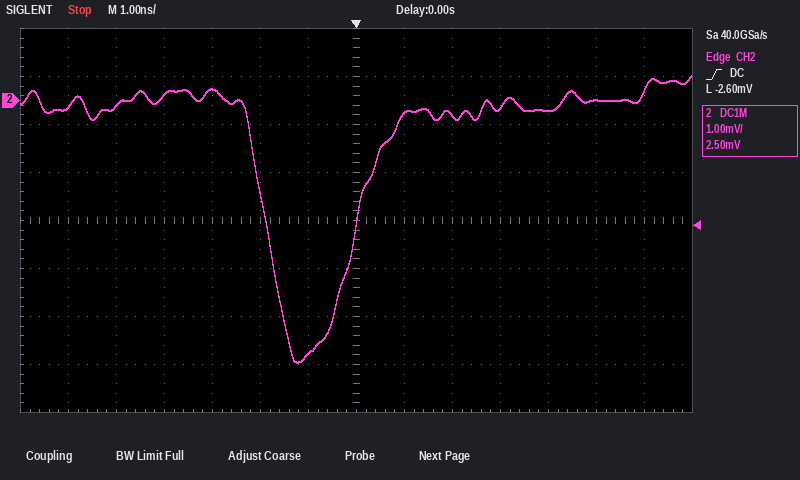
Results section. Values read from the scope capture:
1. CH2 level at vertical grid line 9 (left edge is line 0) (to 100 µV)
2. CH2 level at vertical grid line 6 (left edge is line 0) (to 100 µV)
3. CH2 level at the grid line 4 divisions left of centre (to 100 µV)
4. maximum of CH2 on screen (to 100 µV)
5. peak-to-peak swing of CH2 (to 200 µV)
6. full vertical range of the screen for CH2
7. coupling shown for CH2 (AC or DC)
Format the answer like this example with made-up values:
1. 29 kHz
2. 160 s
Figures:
1. -300 µV
2. -5.3 mV
3. 100 µV
4. 500 µV
5. 6.0 mV
6. 8 mV
7. DC
